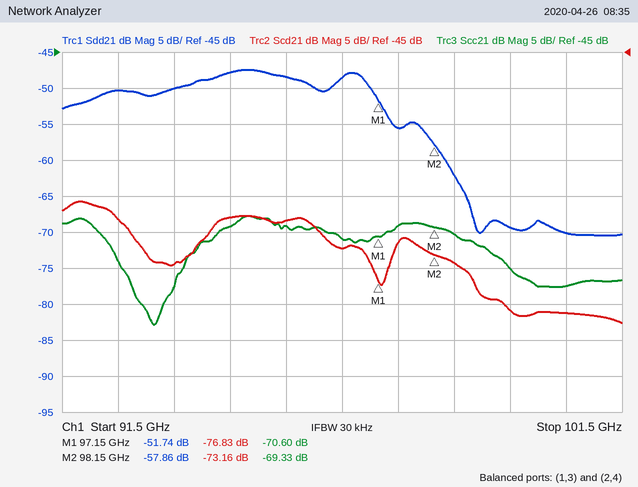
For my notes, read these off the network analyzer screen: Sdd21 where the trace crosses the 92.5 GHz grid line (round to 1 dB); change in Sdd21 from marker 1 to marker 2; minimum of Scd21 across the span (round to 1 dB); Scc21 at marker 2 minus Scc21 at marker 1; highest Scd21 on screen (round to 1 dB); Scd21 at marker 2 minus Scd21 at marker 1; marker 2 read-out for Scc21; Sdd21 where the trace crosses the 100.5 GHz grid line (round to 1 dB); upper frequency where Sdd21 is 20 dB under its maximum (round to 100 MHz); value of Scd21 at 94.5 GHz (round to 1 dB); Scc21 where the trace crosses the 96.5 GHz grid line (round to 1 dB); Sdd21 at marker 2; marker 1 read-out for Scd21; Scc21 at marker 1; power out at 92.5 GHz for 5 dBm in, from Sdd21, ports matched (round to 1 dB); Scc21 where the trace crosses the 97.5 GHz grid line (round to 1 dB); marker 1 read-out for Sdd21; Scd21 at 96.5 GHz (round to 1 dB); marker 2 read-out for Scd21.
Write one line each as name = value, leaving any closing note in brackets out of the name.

Sdd21 where the trace crosses the 92.5 GHz grid line = -50 dB
change in Sdd21 from marker 1 to marker 2 = -6.12 dB
minimum of Scd21 across the span = -83 dB
Scc21 at marker 2 minus Scc21 at marker 1 = 1.27 dB
highest Scd21 on screen = -66 dB
Scd21 at marker 2 minus Scd21 at marker 1 = 3.67 dB
marker 2 read-out for Scc21 = -69.33 dB
Sdd21 where the trace crosses the 100.5 GHz grid line = -70 dB
upper frequency where Sdd21 is 20 dB under its maximum = 98.8 GHz
value of Scd21 at 94.5 GHz = -68 dB
Scc21 where the trace crosses the 96.5 GHz grid line = -71 dB
Sdd21 at marker 2 = -57.86 dB
marker 1 read-out for Scd21 = -76.83 dB
Scc21 at marker 1 = -70.60 dB
power out at 92.5 GHz for 5 dBm in, from Sdd21, ports matched = -45 dBm
Scc21 where the trace crosses the 97.5 GHz grid line = -69 dB
marker 1 read-out for Sdd21 = -51.74 dB
Scd21 at 96.5 GHz = -72 dB
marker 2 read-out for Scd21 = -73.16 dB
